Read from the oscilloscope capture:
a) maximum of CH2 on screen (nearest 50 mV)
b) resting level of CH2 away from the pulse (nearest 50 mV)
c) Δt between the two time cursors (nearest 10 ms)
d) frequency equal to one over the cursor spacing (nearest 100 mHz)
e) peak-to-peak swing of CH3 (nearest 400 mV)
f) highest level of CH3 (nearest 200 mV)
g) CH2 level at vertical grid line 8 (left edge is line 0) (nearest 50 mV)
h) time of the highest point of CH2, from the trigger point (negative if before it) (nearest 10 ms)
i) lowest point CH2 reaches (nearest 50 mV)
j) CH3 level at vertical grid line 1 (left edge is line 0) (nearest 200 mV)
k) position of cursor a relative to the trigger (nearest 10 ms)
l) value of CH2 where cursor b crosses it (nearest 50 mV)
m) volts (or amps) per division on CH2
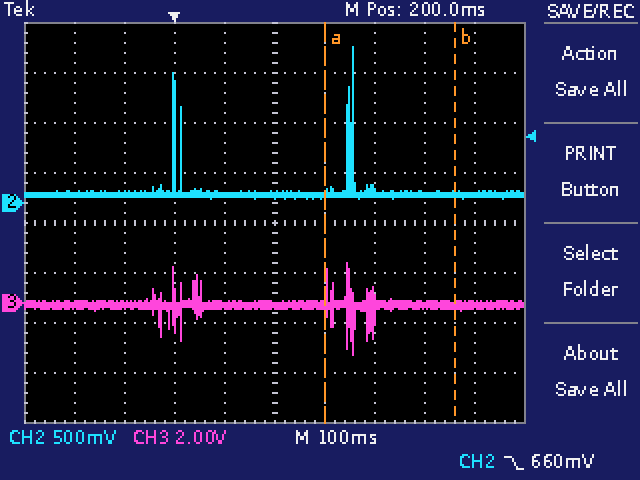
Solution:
1.55 V
100 mV
260 ms
3.8 Hz
3.6 V
1.6 V
100 mV
+360 ms
50 mV
0.0 V
+300 ms
100 mV
500 mV
